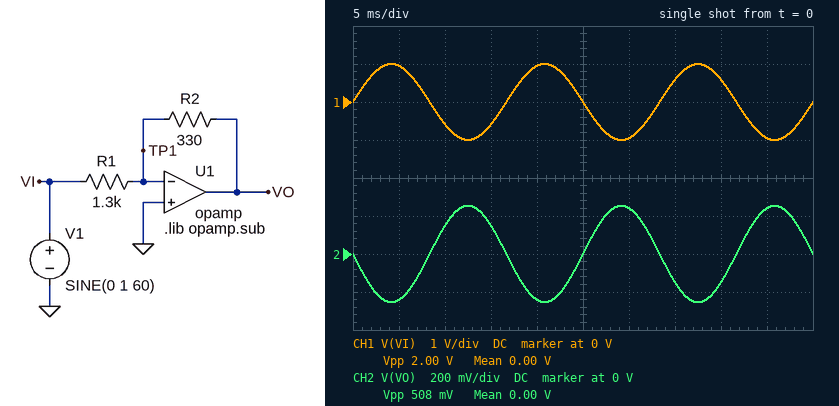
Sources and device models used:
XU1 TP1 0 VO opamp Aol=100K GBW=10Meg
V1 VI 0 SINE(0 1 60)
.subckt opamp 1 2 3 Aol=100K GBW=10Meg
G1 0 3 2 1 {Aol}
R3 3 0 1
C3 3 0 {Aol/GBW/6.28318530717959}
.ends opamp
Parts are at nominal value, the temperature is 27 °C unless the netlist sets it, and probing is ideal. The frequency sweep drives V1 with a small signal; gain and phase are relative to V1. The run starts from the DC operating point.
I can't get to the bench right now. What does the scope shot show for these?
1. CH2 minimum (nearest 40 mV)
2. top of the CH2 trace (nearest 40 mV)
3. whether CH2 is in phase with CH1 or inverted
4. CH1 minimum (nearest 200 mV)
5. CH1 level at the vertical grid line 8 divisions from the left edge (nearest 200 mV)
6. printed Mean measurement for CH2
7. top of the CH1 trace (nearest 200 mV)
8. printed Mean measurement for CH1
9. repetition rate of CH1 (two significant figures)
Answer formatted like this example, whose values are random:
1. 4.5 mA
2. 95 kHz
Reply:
1. -240 mV
2. 240 mV
3. inverted
4. -1.0 V
5. 600 mV
6. 0.00 V
7. 1.0 V
8. 0.00 V
9. 60 Hz
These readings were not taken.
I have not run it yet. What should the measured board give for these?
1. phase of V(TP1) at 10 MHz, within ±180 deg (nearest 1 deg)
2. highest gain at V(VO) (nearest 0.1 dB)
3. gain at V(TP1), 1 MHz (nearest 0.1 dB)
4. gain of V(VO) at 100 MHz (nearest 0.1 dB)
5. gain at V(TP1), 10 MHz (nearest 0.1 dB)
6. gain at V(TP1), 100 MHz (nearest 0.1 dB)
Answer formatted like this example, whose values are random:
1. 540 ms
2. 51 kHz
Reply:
1. 39 deg
2. -11.9 dB
3. -32.0 dB
4. -33.9 dB
5. -16.0 dB
6. -13.9 dB
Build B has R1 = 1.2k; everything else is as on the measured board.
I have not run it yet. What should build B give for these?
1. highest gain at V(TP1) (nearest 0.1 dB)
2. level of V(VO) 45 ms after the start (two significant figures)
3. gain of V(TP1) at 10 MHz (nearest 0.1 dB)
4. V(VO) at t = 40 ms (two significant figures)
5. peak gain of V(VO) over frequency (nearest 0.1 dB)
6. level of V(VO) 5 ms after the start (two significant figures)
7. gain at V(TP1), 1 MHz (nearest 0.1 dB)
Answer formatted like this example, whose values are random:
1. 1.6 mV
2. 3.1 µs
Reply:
1. -13.3 dB
2. 260 mV
3. -15.4 dB
4. -160 mV
5. -11.2 dB
6. -260 mV
7. -31.3 dB
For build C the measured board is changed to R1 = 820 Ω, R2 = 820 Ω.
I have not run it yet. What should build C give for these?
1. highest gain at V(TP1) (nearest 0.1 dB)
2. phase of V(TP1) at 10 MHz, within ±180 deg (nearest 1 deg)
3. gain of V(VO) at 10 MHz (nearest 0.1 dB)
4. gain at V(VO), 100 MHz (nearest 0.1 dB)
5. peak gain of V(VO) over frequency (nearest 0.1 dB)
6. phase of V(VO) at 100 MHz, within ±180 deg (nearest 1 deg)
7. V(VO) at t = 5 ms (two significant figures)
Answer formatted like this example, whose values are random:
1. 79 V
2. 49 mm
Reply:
1. -6.0 dB
2. 27 deg
3. -7.0 dB
4. -26.0 dB
5. 0 dB
6. 93 deg
7. -950 mV
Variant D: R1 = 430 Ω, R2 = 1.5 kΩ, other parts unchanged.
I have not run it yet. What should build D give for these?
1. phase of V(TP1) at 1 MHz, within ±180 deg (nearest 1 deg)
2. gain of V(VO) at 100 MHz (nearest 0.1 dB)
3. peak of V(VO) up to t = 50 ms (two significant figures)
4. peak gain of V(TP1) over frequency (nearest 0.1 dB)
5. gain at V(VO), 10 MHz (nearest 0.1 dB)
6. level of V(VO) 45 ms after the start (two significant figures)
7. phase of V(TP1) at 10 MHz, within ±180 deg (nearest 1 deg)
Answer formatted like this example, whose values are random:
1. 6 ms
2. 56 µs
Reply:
1. 66 deg
2. -22.2 dB
3. 3.5 V
4. -2.2 dB
5. -2.4 dB
6. 3.3 V
7. 13 deg
